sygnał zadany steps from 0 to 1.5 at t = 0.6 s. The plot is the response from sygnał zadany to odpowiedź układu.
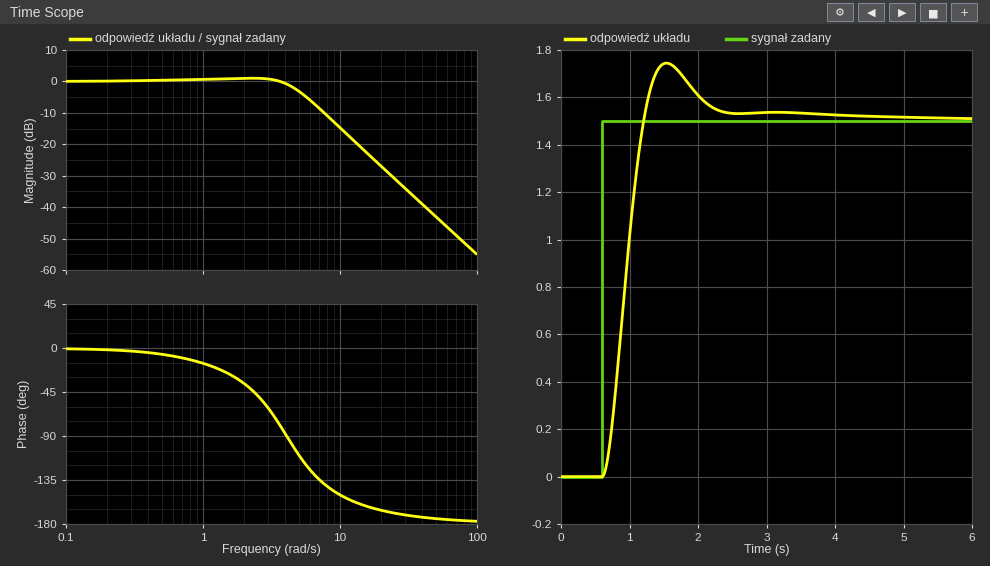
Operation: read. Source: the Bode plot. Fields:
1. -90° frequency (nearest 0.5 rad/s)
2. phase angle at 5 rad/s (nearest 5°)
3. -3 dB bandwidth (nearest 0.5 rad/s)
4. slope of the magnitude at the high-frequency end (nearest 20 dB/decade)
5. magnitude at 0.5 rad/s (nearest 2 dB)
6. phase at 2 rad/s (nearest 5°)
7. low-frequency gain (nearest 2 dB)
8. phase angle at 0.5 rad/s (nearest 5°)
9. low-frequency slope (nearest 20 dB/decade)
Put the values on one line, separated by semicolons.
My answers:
4.0 rad/s; -110°; 5.0 rad/s; -40 dB/decade; 0 dB; -35°; 0 dB; -5°; 0 dB/decade
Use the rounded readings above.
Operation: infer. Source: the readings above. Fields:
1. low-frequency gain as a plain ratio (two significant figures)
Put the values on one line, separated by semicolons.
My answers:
1.0
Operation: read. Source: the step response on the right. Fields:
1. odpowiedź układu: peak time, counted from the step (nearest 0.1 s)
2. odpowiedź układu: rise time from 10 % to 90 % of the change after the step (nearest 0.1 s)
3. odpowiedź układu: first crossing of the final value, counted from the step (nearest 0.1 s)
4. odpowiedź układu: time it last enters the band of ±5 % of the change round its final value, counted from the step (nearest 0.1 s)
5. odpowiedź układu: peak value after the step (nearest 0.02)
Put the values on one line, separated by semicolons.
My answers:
0.9 s; 0.4 s; 0.6 s; 1.5 s; 1.74
